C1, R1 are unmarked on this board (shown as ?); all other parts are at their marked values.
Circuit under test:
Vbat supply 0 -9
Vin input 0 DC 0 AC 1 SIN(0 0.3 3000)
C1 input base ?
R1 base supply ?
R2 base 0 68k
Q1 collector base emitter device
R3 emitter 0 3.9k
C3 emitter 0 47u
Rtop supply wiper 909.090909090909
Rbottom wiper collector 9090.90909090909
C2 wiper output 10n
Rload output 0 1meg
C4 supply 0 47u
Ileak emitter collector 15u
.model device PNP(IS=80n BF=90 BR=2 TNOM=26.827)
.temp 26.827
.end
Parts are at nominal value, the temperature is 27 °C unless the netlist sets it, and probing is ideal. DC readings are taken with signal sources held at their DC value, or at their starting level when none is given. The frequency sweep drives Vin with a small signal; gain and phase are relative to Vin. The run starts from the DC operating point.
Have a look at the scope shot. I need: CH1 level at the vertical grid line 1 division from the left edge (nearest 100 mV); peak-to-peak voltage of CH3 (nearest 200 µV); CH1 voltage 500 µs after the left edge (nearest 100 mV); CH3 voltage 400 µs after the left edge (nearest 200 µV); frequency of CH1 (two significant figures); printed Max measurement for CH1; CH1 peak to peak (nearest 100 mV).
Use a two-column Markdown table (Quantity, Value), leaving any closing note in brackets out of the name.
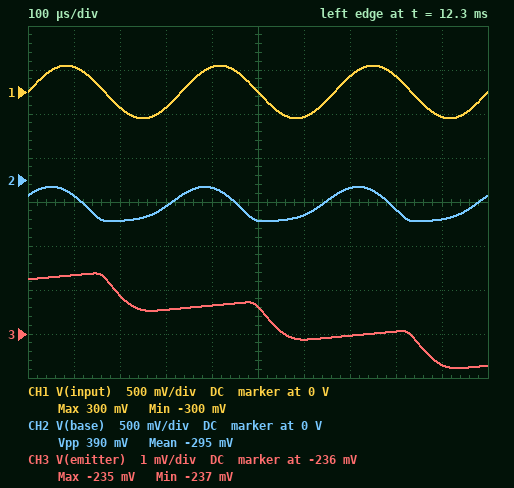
| Quantity | Value |
|---|---|
| CH1 level at the vertical grid line 1 division from the left edge | 300 mV |
| peak-to-peak voltage of CH3 | 2.2 mV |
| CH1 voltage 500 µs after the left edge | 0 V |
| CH3 voltage 400 µs after the left edge | -235.4 mV |
| frequency of CH1 | 3.0 kHz |
| printed Max measurement for CH1 | 300 mV |
| CH1 peak to peak | 600 mV |
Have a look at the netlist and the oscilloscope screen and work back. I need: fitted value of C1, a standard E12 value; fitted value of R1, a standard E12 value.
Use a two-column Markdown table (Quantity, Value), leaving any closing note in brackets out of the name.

| Quantity | Value |
|---|---|
| fitted value of C1, a standard E12 value | 1.5 nF |
| fitted value of R1, a standard E12 value | 1.5 MΩ |
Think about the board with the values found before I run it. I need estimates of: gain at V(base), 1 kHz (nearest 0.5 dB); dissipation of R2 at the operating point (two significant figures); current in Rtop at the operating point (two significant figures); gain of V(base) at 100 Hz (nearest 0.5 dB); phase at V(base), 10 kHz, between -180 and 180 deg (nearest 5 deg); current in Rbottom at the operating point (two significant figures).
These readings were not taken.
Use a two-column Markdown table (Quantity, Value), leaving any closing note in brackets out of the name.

| Quantity | Value |
|---|---|
| gain at V(base), 1 kHz | -11.0 dB |
| dissipation of R2 at the operating point | 2.0 µW |
| current in Rtop at the operating point | 53 µA |
| gain of V(base) at 100 Hz | -30.5 dB |
| phase at V(base), 10 kHz, between -180 and 180 deg | 20 deg |
| current in Rbottom at the operating point | 53 µA |
